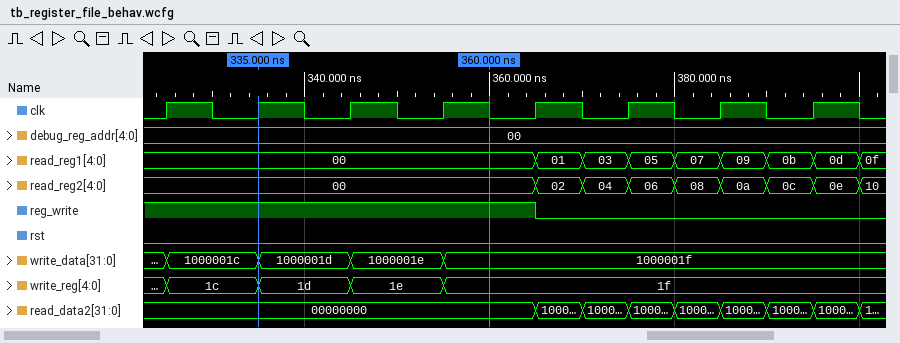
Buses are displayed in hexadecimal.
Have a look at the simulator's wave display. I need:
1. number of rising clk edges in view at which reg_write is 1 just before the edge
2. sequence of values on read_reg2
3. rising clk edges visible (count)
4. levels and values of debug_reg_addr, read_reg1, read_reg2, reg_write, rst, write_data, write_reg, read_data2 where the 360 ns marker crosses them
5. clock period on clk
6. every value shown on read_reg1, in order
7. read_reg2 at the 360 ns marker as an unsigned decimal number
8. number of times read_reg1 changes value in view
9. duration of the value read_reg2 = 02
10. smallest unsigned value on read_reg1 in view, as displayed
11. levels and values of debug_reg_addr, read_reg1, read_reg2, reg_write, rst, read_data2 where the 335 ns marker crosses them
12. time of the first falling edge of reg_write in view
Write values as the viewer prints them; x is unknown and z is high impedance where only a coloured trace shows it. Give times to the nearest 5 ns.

5
00, 02, 04, 06, 08, 0a, 0c, 0e, 10
8
debug_reg_addr=00, read_reg1=00, read_reg2=00, reg_write=1, rst=0, write_data=1000001f, write_reg=1f, read_data2=00000000
10 ns
00, 01, 03, 05, 07, 09, 0b, 0d, 0f
0
8
5 ns
00
debug_reg_addr=00, read_reg1=00, read_reg2=00, reg_write=1, rst=0, read_data2=00000000
365 ns
